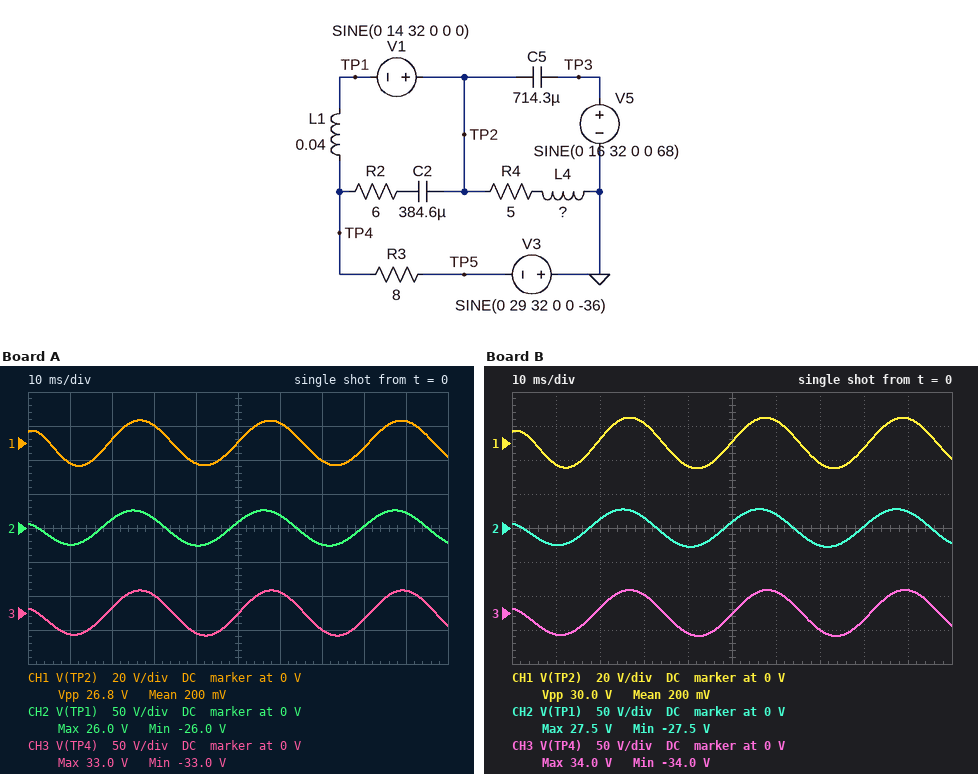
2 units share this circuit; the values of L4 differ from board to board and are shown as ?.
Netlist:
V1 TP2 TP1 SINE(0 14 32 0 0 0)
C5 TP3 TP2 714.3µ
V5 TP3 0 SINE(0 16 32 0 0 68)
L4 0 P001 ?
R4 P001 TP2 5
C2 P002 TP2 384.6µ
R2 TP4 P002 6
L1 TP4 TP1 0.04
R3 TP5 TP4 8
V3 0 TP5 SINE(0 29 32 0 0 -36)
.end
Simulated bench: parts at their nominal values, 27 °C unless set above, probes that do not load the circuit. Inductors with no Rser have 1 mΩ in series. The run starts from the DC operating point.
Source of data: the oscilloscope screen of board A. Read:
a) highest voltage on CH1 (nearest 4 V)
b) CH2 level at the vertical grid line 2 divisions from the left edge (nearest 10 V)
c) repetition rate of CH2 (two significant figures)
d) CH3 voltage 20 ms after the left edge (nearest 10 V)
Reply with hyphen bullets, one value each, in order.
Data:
- 12 V
- 10 V
- 32 Hz
- 10 V
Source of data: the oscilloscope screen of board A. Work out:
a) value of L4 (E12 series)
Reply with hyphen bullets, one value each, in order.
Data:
- 18 mH
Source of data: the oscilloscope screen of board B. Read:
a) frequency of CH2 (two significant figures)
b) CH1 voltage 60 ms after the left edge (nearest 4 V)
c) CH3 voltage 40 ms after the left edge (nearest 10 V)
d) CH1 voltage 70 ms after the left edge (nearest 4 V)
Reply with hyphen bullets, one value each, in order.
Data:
- 32 Hz
- 12 V
- -30 V
- -12 V
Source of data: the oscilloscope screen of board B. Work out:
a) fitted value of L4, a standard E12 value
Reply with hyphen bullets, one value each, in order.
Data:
- 22 mH
